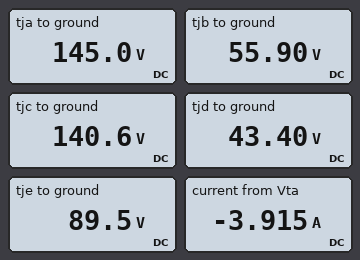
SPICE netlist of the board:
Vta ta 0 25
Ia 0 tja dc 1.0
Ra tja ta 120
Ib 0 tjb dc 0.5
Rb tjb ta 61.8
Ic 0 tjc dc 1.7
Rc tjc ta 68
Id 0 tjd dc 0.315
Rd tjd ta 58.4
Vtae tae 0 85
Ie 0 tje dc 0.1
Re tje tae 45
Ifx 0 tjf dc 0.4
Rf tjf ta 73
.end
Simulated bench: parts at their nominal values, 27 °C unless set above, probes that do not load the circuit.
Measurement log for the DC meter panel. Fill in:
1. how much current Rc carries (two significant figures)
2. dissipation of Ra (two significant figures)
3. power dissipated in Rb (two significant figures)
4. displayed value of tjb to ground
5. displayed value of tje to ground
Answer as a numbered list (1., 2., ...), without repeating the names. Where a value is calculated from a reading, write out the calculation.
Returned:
1. (140.6 V - 25 V) / 68 Ω = 1.7 A
2. (145 V - 25 V)^2 / 120 Ω = 120 W
3. (55.9 V - 25 V)^2 / 61.8 Ω = 15 W
4. 55.90 V
5. 89.5 V
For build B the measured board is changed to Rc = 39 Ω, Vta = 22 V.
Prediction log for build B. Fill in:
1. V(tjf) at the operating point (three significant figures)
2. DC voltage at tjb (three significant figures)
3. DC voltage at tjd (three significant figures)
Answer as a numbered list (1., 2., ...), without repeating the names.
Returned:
1. 51.2 V
2. 52.9 V
3. 40.4 V
